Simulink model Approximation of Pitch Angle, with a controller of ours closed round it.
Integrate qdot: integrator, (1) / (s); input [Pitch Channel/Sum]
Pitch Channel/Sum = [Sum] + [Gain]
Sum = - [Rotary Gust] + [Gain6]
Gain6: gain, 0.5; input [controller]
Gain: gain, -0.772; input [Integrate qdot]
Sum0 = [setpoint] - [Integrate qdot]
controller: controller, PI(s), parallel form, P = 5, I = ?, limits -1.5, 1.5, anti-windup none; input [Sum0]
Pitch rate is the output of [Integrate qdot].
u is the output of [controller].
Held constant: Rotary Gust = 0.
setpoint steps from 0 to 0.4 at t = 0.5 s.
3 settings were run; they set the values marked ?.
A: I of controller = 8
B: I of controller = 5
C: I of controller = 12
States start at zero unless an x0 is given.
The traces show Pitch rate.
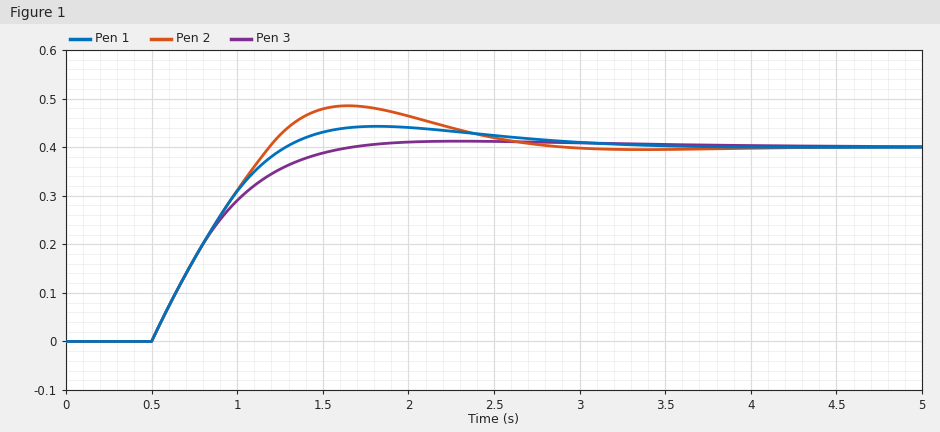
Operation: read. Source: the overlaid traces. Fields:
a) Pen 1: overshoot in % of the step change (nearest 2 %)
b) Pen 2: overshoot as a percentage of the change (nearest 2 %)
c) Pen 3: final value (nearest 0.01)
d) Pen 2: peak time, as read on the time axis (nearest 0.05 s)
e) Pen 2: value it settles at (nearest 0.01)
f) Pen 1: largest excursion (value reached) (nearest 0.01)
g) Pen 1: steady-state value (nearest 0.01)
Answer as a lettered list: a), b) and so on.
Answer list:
a) 10 %
b) 22 %
c) 0.40
d) 1.65 s
e) 0.40
f) 0.44
g) 0.40
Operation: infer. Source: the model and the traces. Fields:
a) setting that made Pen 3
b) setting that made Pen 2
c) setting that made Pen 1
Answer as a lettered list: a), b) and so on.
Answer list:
a) B
b) C
c) A
